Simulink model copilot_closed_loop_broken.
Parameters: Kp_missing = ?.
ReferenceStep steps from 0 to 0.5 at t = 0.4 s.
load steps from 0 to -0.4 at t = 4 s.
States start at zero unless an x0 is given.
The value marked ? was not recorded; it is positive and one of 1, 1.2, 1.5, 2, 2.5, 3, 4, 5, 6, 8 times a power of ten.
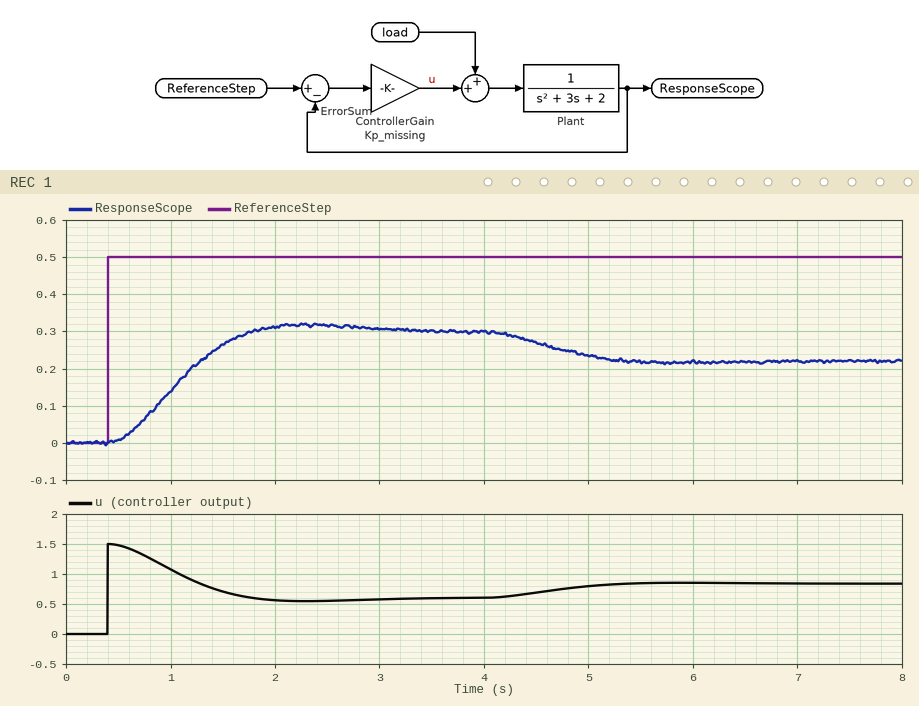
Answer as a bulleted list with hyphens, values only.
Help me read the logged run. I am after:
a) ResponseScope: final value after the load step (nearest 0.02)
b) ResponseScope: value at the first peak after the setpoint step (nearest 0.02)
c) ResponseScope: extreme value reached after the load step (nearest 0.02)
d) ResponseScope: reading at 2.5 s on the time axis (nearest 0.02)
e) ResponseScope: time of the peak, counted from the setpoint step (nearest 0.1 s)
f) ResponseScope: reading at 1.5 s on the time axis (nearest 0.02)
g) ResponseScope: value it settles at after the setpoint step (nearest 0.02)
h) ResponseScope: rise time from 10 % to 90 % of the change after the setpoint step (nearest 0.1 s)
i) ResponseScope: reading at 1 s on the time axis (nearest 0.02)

- 0.22
- 0.32
- 0.22
- 0.32
- 1.9 s
- 0.26
- 0.30
- 0.9 s
- 0.14
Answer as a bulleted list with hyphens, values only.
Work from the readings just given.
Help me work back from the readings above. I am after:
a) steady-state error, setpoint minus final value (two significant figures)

- 0.20
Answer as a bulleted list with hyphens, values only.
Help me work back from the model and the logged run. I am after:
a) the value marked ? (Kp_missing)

- 3
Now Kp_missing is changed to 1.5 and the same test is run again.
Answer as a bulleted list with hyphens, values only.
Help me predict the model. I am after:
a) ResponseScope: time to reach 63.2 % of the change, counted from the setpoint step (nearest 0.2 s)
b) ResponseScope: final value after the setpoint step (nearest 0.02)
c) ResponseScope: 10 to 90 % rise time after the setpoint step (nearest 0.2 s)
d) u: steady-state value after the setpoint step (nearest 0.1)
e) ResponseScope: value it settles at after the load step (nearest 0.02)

- 1.0 s
- 0.22
- 1.4 s
- 0.4
- 0.10
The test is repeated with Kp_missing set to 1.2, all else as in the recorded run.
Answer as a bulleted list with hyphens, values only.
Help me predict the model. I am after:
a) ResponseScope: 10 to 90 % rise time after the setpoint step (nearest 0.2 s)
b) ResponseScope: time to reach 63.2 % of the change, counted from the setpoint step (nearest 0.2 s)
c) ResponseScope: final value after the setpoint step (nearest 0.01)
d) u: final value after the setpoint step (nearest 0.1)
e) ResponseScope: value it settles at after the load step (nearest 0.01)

- 1.4 s
- 1.0 s
- 0.19
- 0.4
- 0.06
